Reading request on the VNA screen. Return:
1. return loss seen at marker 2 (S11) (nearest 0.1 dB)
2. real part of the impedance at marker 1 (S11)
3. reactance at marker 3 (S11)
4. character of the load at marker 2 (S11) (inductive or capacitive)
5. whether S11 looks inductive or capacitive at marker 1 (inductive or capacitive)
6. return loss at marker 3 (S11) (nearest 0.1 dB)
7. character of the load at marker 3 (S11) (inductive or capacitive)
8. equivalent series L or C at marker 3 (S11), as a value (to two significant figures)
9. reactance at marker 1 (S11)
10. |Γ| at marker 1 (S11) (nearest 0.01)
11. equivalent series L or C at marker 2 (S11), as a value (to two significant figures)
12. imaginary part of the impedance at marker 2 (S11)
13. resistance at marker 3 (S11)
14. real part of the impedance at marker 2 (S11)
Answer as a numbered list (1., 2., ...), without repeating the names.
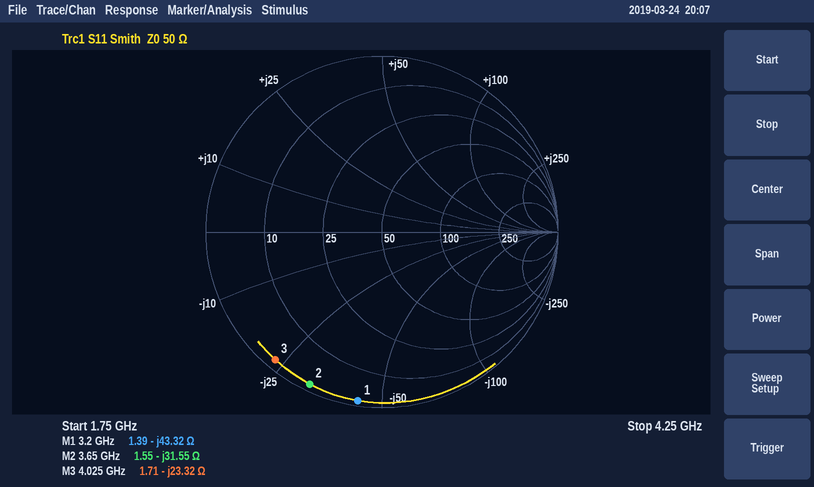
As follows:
1. 0.4 dB
2. 1.39 Ω
3. -23.32 Ω
4. capacitive
5. capacitive
6. 0.5 dB
7. capacitive
8. 1.7 pF
9. -43.32 Ω
10. 0.97
11. 1.4 pF
12. -31.55 Ω
13. 1.71 Ω
14. 1.55 Ω
